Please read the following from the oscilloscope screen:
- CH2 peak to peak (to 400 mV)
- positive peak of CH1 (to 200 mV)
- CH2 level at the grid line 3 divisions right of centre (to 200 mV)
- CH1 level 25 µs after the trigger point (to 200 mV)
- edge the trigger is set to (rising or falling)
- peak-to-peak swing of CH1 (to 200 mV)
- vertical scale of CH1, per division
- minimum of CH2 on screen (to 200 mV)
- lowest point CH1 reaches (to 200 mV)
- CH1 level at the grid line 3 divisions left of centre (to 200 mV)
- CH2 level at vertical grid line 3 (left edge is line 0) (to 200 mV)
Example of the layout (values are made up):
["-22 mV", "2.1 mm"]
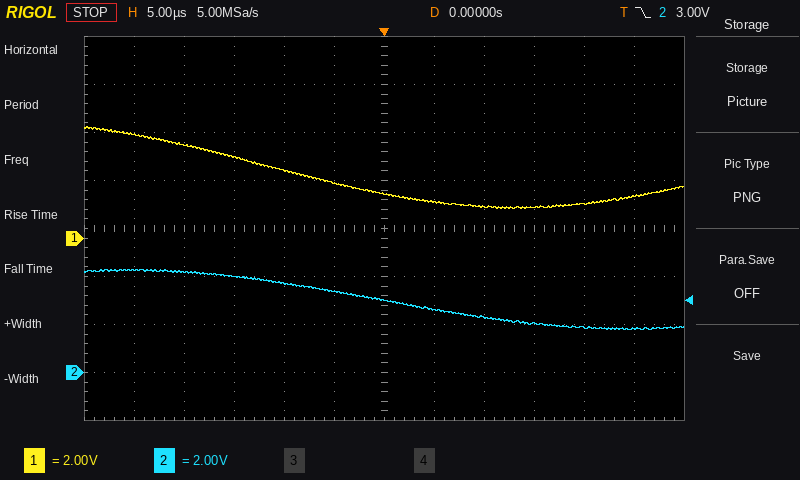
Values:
["2.4 V", "4.6 V", "2.0 V", "1.8 V", "falling", "3.4 V", "2 V", "1.8 V", "1.2 V", "3.4 V", "4.0 V"]
